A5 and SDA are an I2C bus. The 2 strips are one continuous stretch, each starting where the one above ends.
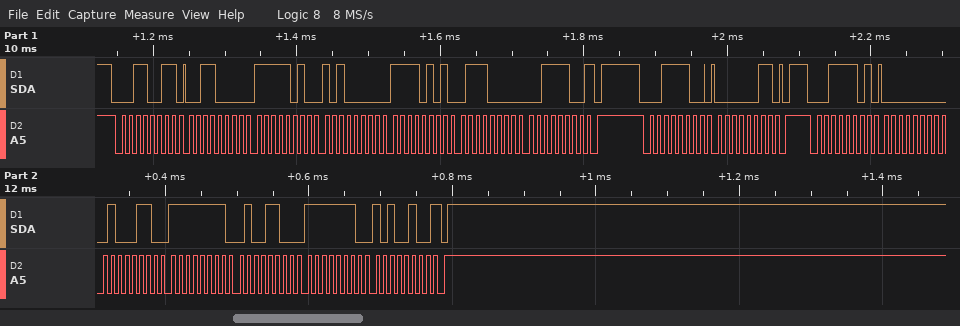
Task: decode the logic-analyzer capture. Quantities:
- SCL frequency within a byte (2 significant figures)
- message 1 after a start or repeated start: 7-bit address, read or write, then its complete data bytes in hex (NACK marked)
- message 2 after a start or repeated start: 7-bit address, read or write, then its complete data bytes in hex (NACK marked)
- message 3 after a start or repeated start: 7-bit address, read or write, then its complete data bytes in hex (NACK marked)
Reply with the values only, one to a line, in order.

100 kHz
0x19 read: 30 FA A0 F5 70 3C NACK
0x1E write: 03
0x1E read: 00 46 FF 4C FE A4 NACK
